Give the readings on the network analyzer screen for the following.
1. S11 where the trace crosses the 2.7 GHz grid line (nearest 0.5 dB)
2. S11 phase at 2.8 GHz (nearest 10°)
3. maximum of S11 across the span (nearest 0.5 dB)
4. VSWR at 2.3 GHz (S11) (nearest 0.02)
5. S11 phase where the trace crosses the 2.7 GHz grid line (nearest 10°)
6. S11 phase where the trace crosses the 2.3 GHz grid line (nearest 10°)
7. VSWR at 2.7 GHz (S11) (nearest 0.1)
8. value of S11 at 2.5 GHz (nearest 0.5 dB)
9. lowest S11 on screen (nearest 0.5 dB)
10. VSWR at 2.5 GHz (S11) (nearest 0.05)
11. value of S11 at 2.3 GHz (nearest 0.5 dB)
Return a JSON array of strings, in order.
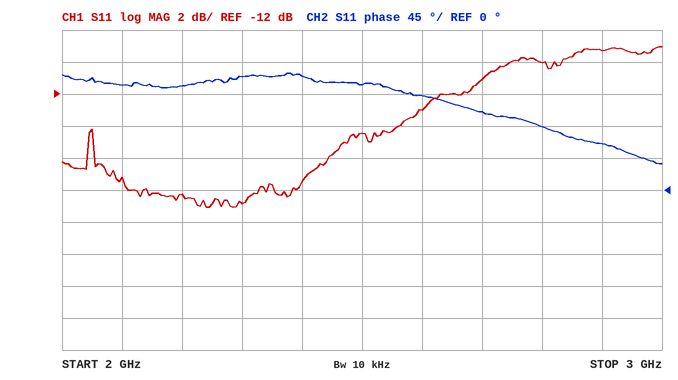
["-11.0 dB", "90°", "-9.0 dB", "1.26", "110°", "160°", "1.8", "-14.5 dB", "-19.0 dB", "1.45", "-19.0 dB"]
